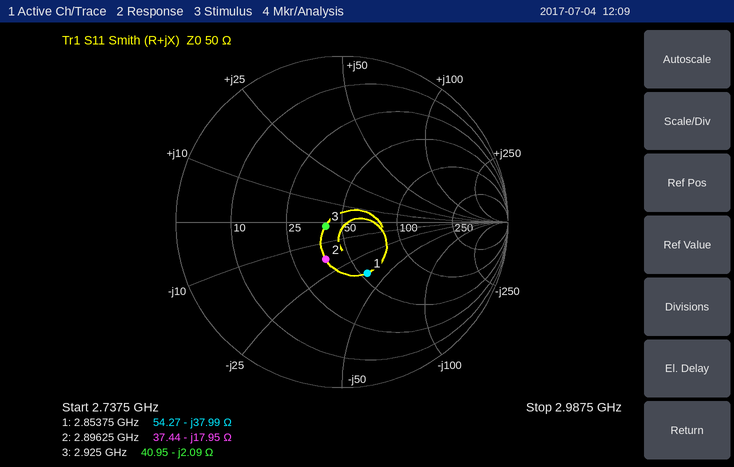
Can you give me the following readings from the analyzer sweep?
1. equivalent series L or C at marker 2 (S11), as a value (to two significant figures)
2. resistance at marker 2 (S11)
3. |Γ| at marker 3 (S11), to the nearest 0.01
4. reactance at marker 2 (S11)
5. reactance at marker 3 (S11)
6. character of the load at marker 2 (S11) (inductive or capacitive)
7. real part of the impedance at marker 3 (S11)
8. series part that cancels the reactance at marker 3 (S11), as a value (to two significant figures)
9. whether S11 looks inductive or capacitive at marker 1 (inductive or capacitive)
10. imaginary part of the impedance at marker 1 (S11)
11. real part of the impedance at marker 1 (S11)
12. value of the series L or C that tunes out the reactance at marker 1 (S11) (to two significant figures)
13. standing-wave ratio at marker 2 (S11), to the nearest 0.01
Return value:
3.1 pF
37.44 Ω
0.10
-17.95 Ω
-2.09 Ω
capacitive
40.95 Ω
110 pH
capacitive
-37.99 Ω
54.27 Ω
2.1 nH
1.65
